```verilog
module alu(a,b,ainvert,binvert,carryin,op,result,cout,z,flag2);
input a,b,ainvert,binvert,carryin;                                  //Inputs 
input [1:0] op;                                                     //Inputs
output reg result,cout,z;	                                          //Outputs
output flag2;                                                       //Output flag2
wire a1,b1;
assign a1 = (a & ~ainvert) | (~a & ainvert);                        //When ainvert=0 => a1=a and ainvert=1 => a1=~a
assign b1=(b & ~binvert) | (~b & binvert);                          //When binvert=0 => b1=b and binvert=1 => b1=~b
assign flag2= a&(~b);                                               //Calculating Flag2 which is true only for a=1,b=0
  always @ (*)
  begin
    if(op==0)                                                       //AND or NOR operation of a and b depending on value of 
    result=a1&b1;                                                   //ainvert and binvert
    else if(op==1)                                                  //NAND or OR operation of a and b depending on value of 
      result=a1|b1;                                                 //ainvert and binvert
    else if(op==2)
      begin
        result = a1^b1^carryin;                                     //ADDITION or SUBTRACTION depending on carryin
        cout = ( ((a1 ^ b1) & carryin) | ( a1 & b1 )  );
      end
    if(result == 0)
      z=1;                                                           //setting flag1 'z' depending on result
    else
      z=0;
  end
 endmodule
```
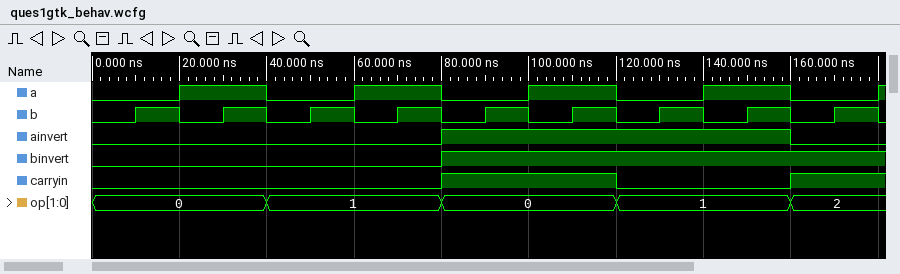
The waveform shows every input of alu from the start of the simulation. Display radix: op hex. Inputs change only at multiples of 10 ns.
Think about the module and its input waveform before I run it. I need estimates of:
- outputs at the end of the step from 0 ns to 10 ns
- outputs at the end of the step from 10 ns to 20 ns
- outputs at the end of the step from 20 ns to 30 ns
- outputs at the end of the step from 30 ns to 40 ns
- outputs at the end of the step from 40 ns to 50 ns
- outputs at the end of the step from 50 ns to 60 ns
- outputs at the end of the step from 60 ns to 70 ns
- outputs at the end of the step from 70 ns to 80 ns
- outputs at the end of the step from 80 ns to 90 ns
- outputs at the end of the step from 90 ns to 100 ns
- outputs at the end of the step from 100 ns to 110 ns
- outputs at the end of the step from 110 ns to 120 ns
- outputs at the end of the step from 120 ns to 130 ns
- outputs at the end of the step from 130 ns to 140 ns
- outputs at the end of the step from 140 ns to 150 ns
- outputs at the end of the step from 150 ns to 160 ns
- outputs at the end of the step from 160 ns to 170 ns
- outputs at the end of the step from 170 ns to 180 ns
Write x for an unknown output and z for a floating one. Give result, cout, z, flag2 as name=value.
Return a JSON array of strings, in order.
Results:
["result=0, cout=x, z=1, flag2=0", "result=0, cout=x, z=1, flag2=0", "result=0, cout=x, z=1, flag2=1", "result=1, cout=x, z=0, flag2=0", "result=0, cout=x, z=1, flag2=0", "result=1, cout=x, z=0, flag2=0", "result=1, cout=x, z=0, flag2=1", "result=1, cout=x, z=0, flag2=0", "result=1, cout=x, z=0, flag2=0", "result=0, cout=x, z=1, flag2=0", "result=0, cout=x, z=1, flag2=1", "result=0, cout=x, z=1, flag2=0", "result=1, cout=x, z=0, flag2=0", "result=1, cout=x, z=0, flag2=0", "result=1, cout=x, z=0, flag2=1", "result=0, cout=x, z=1, flag2=0", "result=0, cout=1, z=1, flag2=0", "result=1, cout=0, z=0, flag2=0"]
